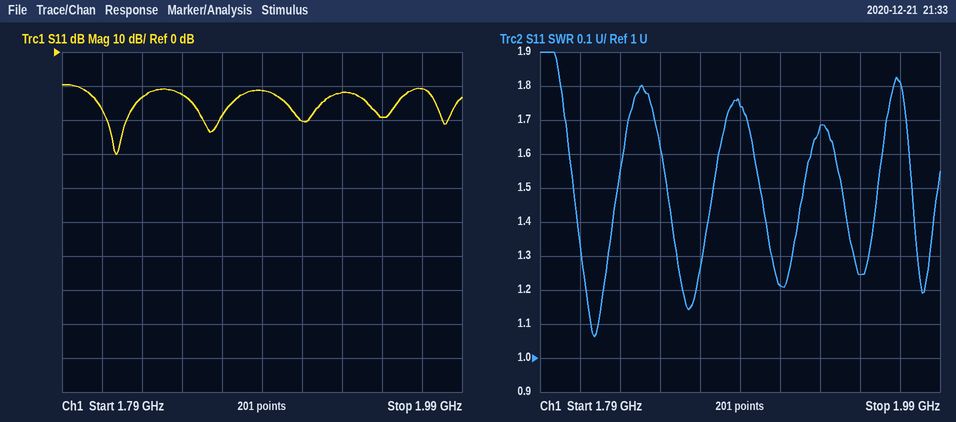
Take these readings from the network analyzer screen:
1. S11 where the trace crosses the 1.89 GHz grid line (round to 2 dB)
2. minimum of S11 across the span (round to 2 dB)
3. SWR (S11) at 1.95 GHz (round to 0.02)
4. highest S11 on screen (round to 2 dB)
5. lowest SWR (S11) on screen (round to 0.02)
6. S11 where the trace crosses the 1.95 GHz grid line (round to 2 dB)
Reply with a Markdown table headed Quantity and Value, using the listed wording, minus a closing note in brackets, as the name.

| Quantity | Value |
|---|---|
| S11 where the trace crosses the 1.89 GHz grid line | -12 dB |
| minimum of S11 across the span | -30 dB |
| SWR (S11) at 1.95 GHz | 1.24 |
| highest S11 on screen | -10 dB |
| lowest SWR (S11) on screen | 1.06 |
| S11 where the trace crosses the 1.95 GHz grid line | -20 dB |
